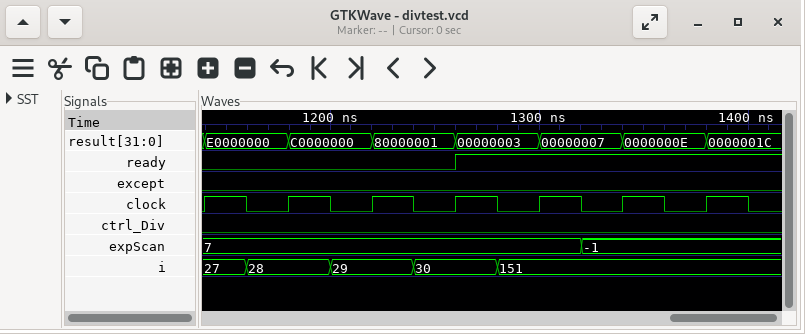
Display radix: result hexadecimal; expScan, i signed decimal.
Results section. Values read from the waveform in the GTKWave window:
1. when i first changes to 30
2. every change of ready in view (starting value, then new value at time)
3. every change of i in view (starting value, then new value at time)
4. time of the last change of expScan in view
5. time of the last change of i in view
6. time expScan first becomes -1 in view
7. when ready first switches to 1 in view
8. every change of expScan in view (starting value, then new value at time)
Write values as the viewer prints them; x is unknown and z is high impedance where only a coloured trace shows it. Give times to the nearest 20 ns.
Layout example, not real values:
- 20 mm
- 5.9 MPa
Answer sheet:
- 1240 ns
- 0, 1 at 1260 ns
- 27, 28 at 1160 ns, 29 at 1200 ns, 30 at 1240 ns, 151 at 1280 ns
- 1320 ns
- 1280 ns
- 1320 ns
- 1260 ns
- 7, -1 at 1320 ns
